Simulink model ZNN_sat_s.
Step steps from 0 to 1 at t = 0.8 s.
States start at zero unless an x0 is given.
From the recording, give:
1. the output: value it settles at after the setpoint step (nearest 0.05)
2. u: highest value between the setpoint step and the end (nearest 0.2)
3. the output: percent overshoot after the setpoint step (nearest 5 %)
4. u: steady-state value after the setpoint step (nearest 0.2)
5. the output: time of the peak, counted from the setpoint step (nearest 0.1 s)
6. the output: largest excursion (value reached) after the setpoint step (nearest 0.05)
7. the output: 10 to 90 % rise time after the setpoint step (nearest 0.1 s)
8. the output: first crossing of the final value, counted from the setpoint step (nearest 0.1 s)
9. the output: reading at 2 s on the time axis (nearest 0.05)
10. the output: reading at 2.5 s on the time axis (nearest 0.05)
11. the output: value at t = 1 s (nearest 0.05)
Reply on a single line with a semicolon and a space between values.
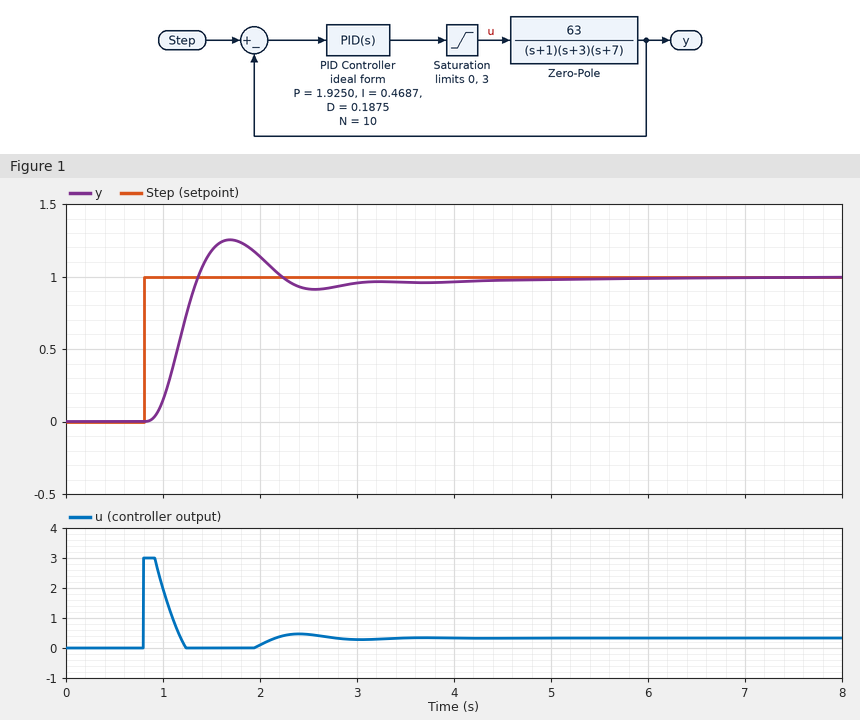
1.00; 3.0; 25 %; 0.4; 0.9 s; 1.25; 0.3 s; 0.6 s; 1.15; 0.90; 0.15
